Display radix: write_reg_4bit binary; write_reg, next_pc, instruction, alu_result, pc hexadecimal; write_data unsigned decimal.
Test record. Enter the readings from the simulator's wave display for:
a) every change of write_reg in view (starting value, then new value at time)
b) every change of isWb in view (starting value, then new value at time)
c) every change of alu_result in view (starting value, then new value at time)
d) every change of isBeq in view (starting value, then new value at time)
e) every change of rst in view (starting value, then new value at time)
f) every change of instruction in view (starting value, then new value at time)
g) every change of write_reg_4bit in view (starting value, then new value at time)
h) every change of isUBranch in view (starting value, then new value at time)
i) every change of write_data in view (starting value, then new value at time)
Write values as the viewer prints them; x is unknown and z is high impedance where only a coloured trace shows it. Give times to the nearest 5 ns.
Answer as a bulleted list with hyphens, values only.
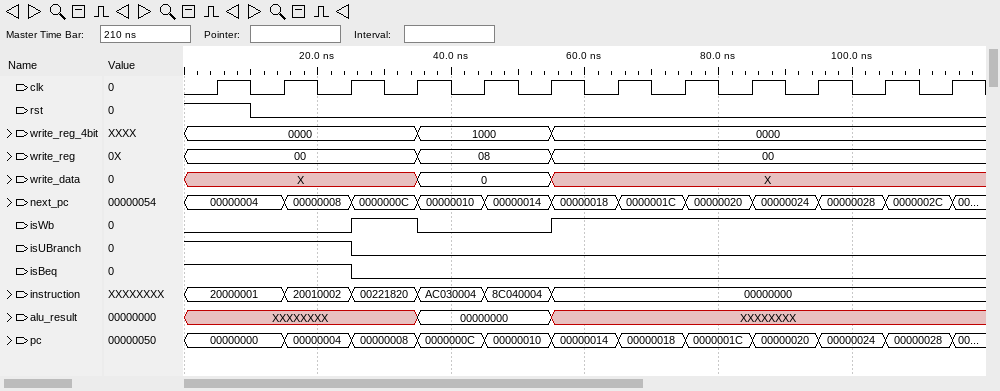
- 00, 08 at 35 ns, 00 at 55 ns
- 0, 1 at 25 ns, 0 at 35 ns, 1 at 55 ns
- XXXXXXXX, 00000000 at 35 ns, XXXXXXXX at 55 ns
- 1, 0 at 25 ns
- 1, 0 at 10 ns
- 20000001, 20010002 at 15 ns, 00221820 at 25 ns, AC030004 at 35 ns, 8C040004 at 45 ns, 00000000 at 55 ns
- 0000, 1000 at 35 ns, 0000 at 55 ns
- 1, 0 at 25 ns
- X, 0 at 35 ns, X at 55 ns
